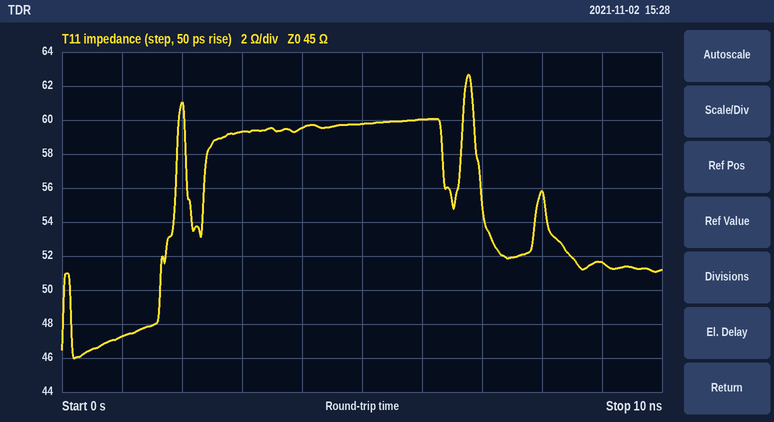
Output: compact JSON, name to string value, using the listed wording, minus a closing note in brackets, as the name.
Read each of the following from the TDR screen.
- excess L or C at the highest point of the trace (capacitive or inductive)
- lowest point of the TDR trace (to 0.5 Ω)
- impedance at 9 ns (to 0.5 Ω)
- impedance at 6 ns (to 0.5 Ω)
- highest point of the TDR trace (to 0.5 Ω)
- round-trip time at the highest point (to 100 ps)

{"excess L or C at the highest point of the trace": "inductive", "lowest point of the TDR trace": "46.0 Ω", "impedance at 9 ns": "51.5 Ω", "impedance at 6 ns": "60.0 Ω", "highest point of the TDR trace": "62.5 Ω", "round-trip time at the highest point": "6.8 ns"}
